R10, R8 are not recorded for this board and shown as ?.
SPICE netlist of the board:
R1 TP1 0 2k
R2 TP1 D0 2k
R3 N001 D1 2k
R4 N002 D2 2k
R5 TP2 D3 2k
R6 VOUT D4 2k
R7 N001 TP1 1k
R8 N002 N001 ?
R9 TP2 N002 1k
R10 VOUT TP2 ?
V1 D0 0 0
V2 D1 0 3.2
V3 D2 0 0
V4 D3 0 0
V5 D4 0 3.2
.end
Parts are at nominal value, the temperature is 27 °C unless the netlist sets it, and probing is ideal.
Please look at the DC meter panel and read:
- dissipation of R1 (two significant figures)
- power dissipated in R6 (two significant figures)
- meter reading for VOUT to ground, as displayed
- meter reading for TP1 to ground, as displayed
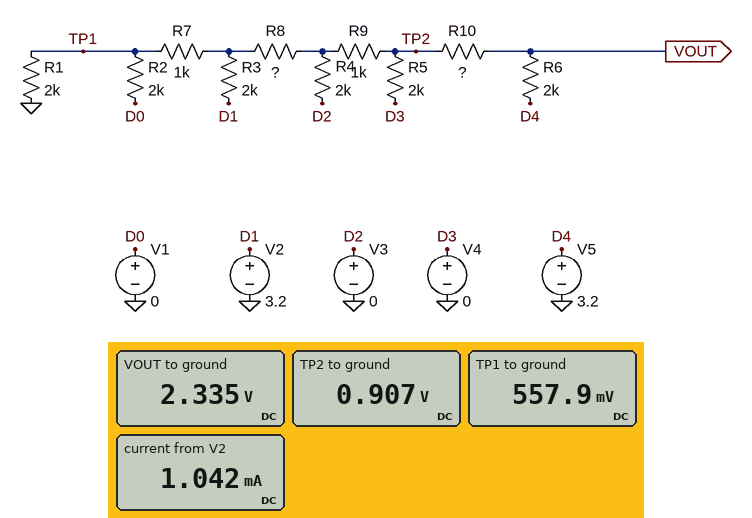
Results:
160 µW
370 µW
2.335 V
557.9 mV
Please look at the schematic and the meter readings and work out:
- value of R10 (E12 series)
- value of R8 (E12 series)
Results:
3.3 kΩ
390 Ω
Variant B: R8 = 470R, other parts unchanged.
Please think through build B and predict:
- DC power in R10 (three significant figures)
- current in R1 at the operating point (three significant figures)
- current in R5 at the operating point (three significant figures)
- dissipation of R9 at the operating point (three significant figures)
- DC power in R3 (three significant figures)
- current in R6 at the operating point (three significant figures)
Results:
623 µW
283 µA
448 µA
190 nW
2.14 mW
435 µA
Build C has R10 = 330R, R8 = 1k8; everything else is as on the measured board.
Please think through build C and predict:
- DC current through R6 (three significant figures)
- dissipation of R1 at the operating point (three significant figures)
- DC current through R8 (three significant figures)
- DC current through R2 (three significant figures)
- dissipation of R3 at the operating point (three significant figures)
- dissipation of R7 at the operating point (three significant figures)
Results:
855 µA
235 µW
229 µA
343 µA
1.67 mW
470 µW
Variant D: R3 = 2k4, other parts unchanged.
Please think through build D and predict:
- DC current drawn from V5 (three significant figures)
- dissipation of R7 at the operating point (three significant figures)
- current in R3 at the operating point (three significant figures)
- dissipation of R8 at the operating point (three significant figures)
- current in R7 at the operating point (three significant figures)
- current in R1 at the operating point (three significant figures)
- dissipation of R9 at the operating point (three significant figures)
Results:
442 µA
253 µW
914 µA
65.8 µW
503 µA
252 µA
154 nW
